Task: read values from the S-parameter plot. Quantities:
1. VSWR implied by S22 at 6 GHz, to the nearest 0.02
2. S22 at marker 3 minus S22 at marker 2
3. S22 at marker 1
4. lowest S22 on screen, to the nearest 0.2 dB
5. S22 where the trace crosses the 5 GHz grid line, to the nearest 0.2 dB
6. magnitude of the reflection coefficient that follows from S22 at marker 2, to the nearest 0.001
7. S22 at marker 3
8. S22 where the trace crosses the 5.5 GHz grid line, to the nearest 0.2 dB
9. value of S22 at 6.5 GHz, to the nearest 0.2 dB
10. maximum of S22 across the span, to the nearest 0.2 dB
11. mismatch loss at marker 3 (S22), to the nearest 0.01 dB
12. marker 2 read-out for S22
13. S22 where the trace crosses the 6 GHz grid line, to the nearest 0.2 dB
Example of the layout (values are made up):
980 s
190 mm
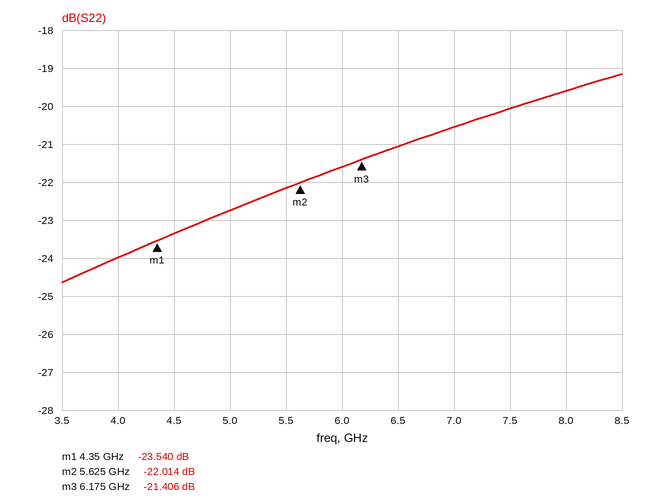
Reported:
1.18
0.608 dB
-23.540 dB
-24.6 dB
-22.8 dB
0.079
-21.406 dB
-22.2 dB
-21.0 dB
-19.2 dB
0.03 dB
-22.014 dB
-21.6 dB
